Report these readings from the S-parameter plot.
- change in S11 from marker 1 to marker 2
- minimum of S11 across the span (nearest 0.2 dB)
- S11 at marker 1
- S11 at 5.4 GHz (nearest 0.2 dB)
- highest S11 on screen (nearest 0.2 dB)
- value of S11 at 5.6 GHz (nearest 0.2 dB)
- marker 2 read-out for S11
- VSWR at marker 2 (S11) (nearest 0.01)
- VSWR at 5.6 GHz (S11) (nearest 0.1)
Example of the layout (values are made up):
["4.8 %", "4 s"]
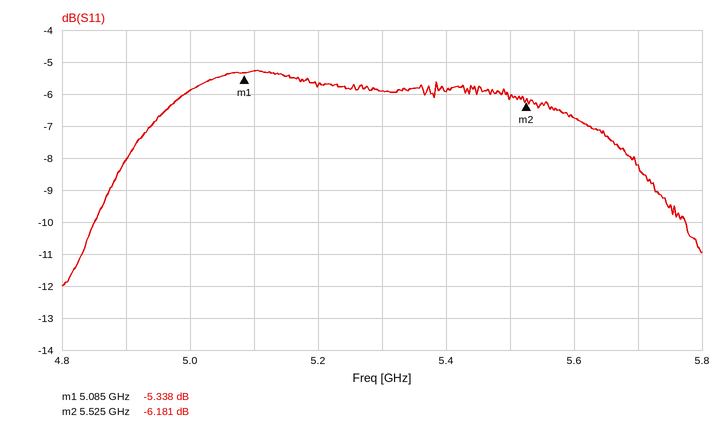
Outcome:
["-0.843 dB", "-12.0 dB", "-5.338 dB", "-6.0 dB", "-5.2 dB", "-6.8 dB", "-6.181 dB", "2.93", "2.7"]
